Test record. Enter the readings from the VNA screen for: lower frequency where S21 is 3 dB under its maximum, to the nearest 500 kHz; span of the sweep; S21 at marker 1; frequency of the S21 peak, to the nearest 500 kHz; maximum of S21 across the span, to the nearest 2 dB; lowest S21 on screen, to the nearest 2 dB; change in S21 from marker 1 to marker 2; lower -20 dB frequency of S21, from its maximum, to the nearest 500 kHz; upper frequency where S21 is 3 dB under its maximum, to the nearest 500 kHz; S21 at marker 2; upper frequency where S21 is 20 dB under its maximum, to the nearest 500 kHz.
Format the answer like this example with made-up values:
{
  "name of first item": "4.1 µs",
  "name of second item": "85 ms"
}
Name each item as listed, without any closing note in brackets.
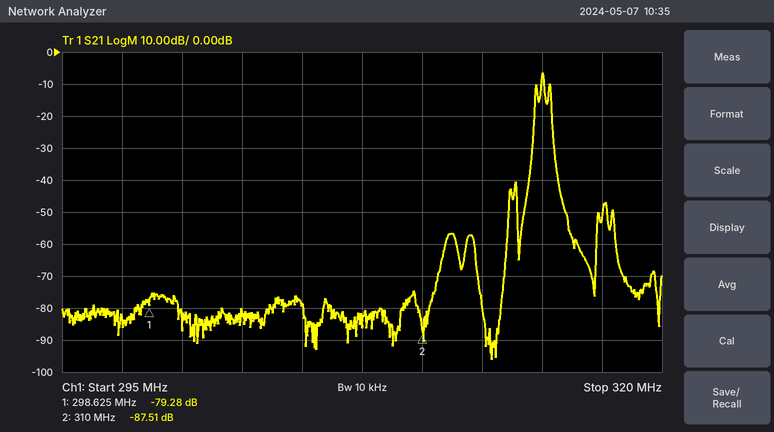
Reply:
{
  "lower frequency where S21 is 3 dB under its maximum, to the nearest 500 kHz": "315.0 MHz",
  "span of the sweep": "25 MHz",
  "S21 at marker 1": "-79.28 dB",
  "frequency of the S21 peak, to the nearest 500 kHz": "315.0 MHz",
  "maximum of S21 across the span, to the nearest 2 dB": "-6 dB",
  "lowest S21 on screen, to the nearest 2 dB": "-96 dB",
  "change in S21 from marker 1 to marker 2": "-8.23 dB",
  "lower -20 dB frequency of S21, from its maximum, to the nearest 500 kHz": "314.5 MHz",
  "upper frequency where S21 is 3 dB under its maximum, to the nearest 500 kHz": "315.0 MHz",
  "S21 at marker 2": "-87.51 dB",
  "upper frequency where S21 is 20 dB under its maximum, to the nearest 500 kHz": "315.5 MHz"
}
